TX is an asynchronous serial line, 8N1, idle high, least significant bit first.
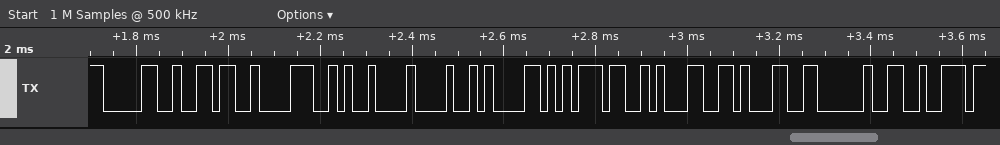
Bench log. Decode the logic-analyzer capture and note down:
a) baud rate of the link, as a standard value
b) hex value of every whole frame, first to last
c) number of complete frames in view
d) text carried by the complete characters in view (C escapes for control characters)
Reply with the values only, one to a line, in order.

57600 baud
0x30 0x36 0x38 0x09 0x48 0x58 0x37 0x31 0x31 0x20 0x72
11
"068\tHX711 r"
